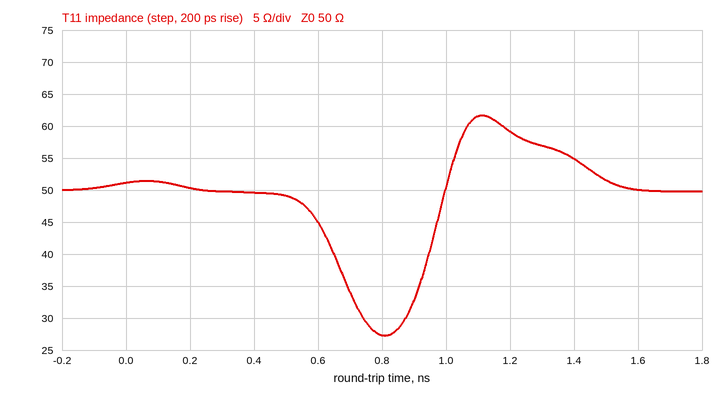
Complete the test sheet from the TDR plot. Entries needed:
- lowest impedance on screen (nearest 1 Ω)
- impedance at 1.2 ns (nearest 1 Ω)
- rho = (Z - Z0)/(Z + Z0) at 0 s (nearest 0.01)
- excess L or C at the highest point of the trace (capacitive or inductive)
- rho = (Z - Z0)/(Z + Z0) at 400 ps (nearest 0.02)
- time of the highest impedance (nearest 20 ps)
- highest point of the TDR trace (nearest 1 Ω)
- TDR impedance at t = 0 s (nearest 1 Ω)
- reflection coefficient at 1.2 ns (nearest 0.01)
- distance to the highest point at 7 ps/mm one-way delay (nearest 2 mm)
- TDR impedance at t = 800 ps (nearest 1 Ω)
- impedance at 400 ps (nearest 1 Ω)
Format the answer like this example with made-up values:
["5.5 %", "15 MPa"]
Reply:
["27 Ω", "59 Ω", "+0.01", "inductive", "0.00", "1.12 ns", "62 Ω", "51 Ω", "+0.08", "80 mm", "27 Ω", "50 Ω"]
